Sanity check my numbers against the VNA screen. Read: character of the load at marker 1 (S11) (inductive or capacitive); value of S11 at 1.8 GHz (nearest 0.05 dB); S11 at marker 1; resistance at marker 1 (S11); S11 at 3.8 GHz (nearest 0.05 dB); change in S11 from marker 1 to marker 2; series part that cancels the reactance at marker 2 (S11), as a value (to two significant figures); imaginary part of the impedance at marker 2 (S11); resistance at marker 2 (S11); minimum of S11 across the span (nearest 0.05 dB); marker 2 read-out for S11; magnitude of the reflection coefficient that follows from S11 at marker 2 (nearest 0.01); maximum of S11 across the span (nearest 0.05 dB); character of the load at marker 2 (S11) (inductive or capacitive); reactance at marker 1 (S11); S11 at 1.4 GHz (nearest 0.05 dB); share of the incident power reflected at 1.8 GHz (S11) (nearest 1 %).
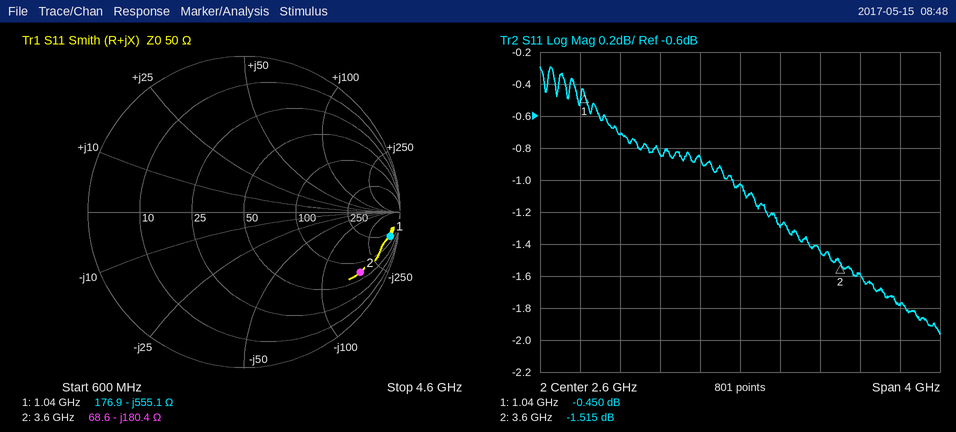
capacitive
-0.85 dB
-0.450 dB
176.9 Ω
-1.60 dB
-1.065 dB
8.0 nH
-180.4 Ω
68.6 Ω
-1.95 dB
-1.515 dB
0.84
-0.30 dB
capacitive
-555.1 Ω
-0.70 dB
82 %
